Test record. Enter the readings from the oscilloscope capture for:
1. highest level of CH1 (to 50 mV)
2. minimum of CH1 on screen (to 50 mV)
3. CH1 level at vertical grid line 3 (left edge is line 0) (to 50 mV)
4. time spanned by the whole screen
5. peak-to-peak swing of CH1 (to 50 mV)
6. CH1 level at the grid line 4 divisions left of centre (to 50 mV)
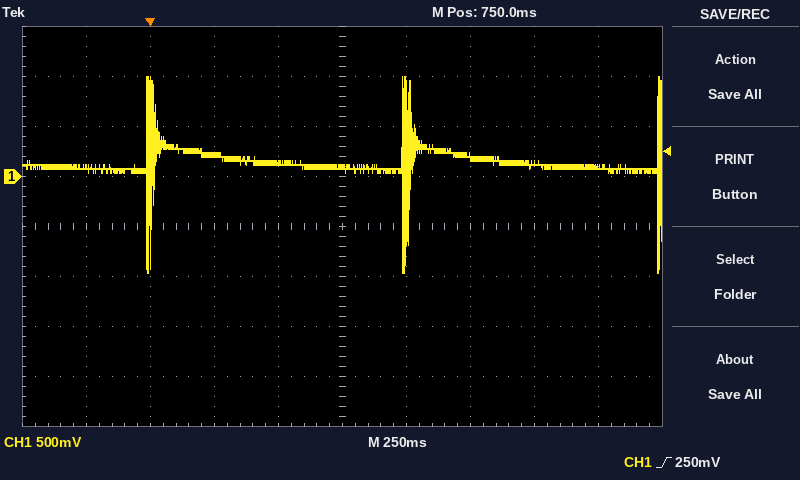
1.00 V
-950 mV
200 mV
2.5 s
1.95 V
100 mV
